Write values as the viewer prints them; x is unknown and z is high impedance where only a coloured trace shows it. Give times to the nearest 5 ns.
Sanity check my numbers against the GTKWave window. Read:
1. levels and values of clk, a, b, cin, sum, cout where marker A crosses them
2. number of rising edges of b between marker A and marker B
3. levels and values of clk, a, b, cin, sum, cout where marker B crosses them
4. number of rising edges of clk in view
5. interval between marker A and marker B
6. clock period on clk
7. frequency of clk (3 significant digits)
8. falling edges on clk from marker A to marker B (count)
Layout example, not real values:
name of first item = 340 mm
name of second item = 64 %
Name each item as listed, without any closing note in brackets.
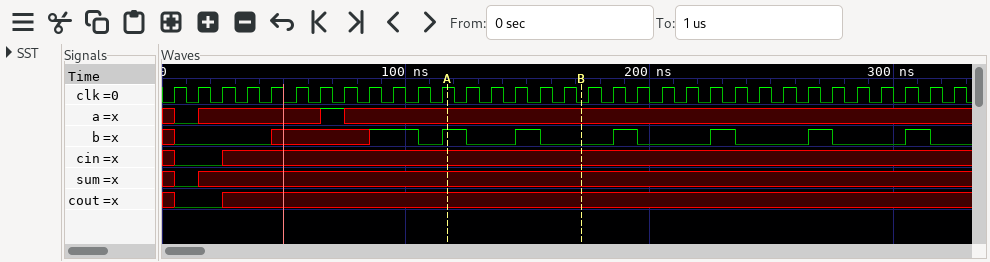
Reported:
levels and values of clk, a, b, cin, sum, cout where marker A crosses them = clk=1, a=x, b=1, cin=x, sum=x, cout=x
number of rising edges of b between marker A and marker B = 1
levels and values of clk, a, b, cin, sum, cout where marker B crosses them = clk=0, a=x, b=0, cin=x, sum=x, cout=x
number of rising edges of clk in view = 33
interval between marker A and marker B = 55 ns
clock period on clk = 10 ns
frequency of clk = 100 MHz
falling edges on clk from marker A to marker B = 6
